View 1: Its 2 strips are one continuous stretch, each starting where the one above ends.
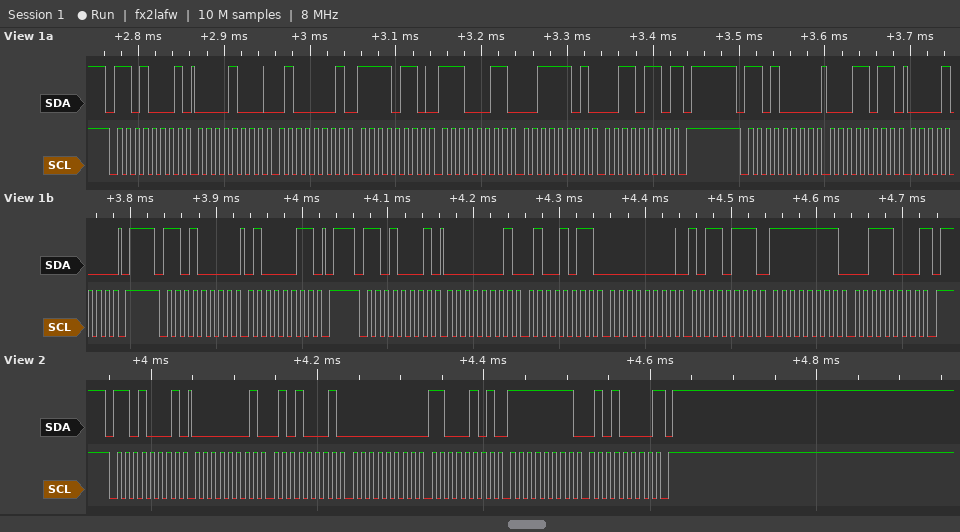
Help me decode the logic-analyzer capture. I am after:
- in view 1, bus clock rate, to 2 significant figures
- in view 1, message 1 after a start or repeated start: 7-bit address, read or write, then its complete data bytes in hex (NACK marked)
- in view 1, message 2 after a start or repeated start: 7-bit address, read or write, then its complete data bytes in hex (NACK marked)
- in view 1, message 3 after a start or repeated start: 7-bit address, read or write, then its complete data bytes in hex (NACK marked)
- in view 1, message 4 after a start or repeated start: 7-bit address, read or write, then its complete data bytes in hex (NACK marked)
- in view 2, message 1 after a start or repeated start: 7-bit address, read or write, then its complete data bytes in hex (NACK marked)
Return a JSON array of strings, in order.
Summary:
["100 kHz", "0x68 read: 08 41 F6 E3 3D 36 NACK", "0x68 write: 1B 08", "0x68 write: 43", "0x68 read: 01 4B 00 B7 FF 38 NACK", "0x68 read: 01 51 00 C5 FF 50 NACK"]
